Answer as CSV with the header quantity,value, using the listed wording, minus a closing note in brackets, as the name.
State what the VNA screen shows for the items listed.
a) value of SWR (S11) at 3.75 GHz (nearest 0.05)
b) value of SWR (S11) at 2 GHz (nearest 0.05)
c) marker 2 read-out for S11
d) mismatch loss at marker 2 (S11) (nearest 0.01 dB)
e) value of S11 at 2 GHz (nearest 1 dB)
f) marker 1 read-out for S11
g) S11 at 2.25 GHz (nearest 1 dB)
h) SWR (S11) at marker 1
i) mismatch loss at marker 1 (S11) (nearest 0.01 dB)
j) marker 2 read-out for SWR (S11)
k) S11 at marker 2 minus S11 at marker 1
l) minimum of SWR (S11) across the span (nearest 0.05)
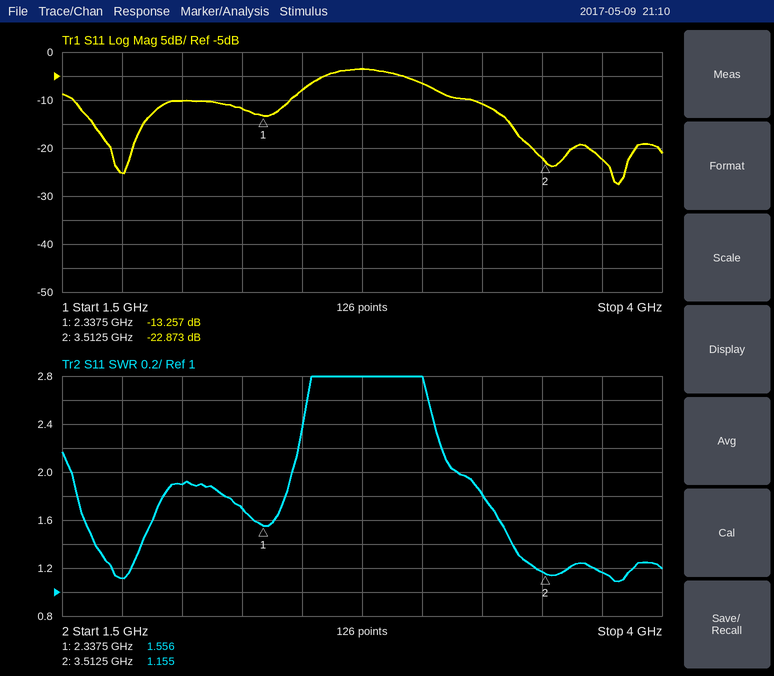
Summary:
quantity,value
value of SWR (S11) at 3.75 GHz,1.15
value of SWR (S11) at 2 GHz,1.90
marker 2 read-out for S11,-22.873 dB
mismatch loss at marker 2 (S11),0.02 dB
value of S11 at 2 GHz,-10 dB
marker 1 read-out for S11,-13.257 dB
S11 at 2.25 GHz,-12 dB
SWR (S11) at marker 1,1.556
mismatch loss at marker 1 (S11),0.21 dB
marker 2 read-out for SWR,1.155
S11 at marker 2 minus S11 at marker 1,-9.616 dB
minimum of SWR (S11) across the span,1.10
